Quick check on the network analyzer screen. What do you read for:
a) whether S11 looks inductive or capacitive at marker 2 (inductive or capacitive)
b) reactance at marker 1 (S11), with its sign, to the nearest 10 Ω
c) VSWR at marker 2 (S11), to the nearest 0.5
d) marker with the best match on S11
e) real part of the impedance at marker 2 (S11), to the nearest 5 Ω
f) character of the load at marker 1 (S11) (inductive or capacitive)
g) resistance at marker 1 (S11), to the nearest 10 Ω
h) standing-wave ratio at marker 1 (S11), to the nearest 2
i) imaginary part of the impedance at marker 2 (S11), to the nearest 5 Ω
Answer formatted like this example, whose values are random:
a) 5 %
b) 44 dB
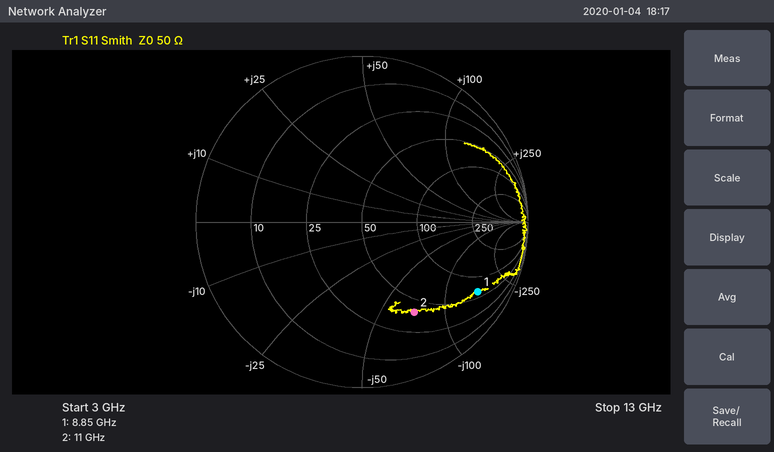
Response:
a) capacitive
b) -160 Ω
c) 4.5
d) marker 2
e) 40 Ω
f) capacitive
g) 60 Ω
h) 10
i) -70 Ω
